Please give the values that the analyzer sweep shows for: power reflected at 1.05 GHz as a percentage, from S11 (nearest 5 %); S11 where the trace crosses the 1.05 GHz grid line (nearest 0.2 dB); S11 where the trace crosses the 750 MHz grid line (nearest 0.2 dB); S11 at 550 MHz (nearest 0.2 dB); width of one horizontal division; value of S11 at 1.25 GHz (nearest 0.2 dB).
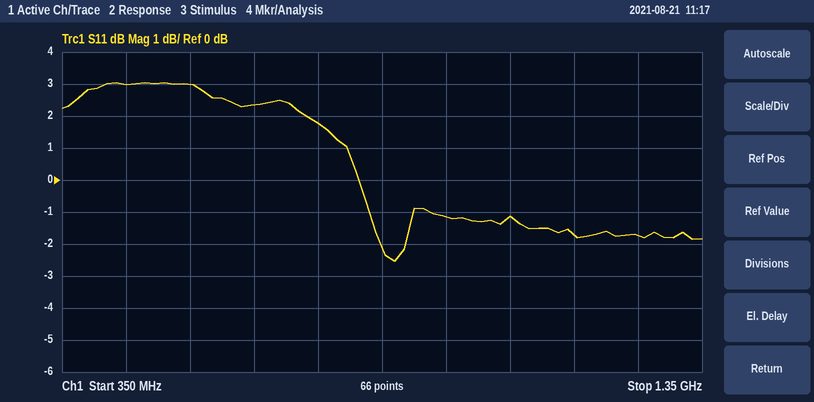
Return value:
75 %
-1.2 dB
1.8 dB
3.0 dB
100 MHz
-1.8 dB
